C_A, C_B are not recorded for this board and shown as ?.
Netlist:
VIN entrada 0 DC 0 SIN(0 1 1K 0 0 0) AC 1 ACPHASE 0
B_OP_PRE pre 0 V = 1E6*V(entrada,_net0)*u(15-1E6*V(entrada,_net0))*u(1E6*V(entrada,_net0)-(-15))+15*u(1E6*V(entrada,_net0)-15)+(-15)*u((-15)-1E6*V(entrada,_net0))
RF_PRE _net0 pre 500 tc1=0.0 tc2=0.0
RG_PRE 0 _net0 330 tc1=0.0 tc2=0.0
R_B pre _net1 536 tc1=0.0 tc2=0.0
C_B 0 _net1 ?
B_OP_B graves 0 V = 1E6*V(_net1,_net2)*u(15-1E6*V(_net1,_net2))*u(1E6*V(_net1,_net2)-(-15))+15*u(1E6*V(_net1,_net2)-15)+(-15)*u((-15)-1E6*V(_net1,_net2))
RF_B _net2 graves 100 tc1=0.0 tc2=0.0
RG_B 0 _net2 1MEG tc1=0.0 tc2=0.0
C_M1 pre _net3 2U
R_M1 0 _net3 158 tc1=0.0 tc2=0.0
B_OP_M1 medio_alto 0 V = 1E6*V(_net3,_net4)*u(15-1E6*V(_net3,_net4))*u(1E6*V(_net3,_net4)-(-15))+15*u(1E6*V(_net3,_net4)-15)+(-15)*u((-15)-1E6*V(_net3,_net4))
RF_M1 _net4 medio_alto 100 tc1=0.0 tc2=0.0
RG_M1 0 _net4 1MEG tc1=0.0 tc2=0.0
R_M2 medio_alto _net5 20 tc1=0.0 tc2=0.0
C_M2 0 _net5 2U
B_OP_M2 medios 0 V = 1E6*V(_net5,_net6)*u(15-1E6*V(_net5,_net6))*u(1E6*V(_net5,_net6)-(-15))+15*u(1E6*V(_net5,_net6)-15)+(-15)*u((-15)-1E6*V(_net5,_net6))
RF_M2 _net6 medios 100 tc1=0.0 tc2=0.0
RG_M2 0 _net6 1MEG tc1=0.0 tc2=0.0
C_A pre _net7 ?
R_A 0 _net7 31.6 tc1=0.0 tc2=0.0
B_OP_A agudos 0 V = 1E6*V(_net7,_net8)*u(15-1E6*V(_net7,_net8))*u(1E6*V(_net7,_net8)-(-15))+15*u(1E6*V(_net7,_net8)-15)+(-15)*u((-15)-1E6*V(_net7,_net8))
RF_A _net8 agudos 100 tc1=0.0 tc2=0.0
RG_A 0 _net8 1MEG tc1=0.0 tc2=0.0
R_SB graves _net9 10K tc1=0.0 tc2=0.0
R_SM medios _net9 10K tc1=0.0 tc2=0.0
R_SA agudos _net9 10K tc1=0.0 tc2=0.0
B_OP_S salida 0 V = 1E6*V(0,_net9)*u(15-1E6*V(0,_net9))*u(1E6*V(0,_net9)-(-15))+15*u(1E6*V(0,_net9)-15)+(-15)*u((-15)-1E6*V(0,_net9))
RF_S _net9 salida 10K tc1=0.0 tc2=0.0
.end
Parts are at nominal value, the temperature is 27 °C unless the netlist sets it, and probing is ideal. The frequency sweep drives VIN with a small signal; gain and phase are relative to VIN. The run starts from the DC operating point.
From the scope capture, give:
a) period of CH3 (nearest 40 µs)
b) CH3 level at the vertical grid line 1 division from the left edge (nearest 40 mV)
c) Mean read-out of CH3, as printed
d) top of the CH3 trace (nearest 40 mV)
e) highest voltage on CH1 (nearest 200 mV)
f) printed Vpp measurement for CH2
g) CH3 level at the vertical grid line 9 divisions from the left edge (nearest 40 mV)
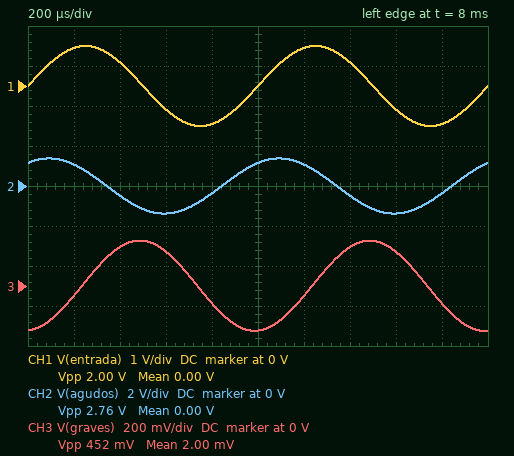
1.00 ms
-40 mV
2.00 mV
240 mV
1.0 V
2.76 V
-80 mV
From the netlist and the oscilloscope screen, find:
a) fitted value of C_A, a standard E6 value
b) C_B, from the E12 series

3.3 µF
3.3 µF
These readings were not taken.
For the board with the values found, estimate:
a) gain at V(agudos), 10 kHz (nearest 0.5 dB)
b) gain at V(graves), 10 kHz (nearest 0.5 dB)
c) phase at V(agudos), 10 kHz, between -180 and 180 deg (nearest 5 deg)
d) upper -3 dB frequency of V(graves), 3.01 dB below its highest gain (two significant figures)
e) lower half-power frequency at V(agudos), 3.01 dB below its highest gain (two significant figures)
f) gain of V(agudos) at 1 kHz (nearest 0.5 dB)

8.0 dB
-33.0 dB
10 deg
90 Hz
1.5 kHz
3.0 dB
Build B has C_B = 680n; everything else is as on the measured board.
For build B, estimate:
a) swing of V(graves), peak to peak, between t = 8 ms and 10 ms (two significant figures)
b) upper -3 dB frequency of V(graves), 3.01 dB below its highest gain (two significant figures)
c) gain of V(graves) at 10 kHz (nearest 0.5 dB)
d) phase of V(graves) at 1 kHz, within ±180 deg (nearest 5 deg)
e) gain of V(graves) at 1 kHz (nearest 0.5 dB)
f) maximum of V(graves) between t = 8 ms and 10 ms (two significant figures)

2.0 V
440 Hz
-19.0 dB
-65 deg
0 dB
1.0 V
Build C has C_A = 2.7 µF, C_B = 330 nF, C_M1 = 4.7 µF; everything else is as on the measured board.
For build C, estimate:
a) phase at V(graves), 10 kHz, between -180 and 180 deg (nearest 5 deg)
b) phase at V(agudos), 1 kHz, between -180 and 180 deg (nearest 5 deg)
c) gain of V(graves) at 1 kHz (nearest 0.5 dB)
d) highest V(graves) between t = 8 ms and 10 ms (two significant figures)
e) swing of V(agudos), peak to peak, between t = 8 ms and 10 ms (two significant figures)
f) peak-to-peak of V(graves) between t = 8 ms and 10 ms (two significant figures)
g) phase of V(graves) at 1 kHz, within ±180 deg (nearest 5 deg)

-85 deg
60 deg
4.5 dB
1.7 V
2.4 V
3.4 V
-50 deg
